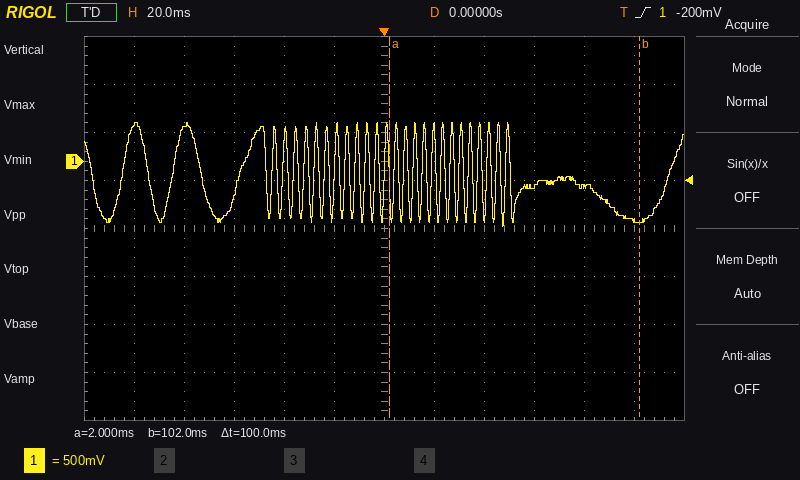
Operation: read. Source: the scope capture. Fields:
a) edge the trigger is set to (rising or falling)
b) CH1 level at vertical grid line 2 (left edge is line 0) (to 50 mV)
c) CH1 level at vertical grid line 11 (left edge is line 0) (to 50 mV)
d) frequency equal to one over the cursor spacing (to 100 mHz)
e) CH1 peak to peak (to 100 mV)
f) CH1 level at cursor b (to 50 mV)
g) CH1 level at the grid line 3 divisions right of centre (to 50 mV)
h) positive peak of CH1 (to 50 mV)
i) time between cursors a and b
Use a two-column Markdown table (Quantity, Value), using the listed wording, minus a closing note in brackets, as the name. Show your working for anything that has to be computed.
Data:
| Quantity | Value |
|---|---|
| edge the trigger is set to | rising |
| CH1 level at vertical grid line 2 (left edge is line 0) | 350 mV |
| CH1 level at vertical grid line 11 (left edge is line 0) | -600 mV |
| frequency equal to one over the cursor spacing | 1 / 100 ms ≈ 10.0 Hz |
| CH1 peak to peak | 1.10 V |
| CH1 level at cursor b | -600 mV |
| CH1 level at the grid line 3 divisions right of centre | -250 mV |
| positive peak of CH1 | 400 mV |
| time between cursors a and b | 100 ms |
